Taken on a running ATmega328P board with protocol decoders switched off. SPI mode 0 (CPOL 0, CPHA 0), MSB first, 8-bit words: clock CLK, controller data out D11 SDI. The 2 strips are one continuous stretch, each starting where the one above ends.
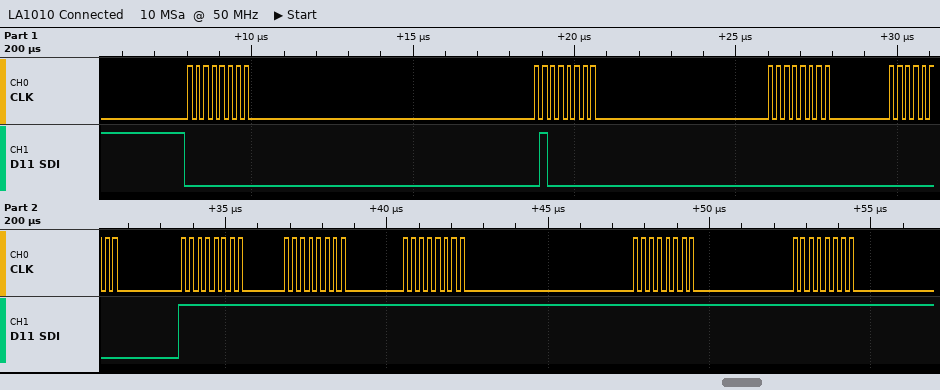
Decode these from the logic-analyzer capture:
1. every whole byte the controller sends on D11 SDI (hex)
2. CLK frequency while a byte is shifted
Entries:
00 40 00 00 FF FF FF FF FF
4 MHz
